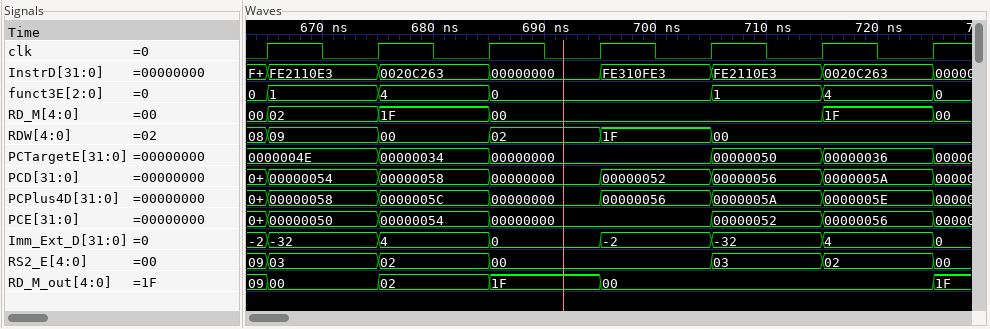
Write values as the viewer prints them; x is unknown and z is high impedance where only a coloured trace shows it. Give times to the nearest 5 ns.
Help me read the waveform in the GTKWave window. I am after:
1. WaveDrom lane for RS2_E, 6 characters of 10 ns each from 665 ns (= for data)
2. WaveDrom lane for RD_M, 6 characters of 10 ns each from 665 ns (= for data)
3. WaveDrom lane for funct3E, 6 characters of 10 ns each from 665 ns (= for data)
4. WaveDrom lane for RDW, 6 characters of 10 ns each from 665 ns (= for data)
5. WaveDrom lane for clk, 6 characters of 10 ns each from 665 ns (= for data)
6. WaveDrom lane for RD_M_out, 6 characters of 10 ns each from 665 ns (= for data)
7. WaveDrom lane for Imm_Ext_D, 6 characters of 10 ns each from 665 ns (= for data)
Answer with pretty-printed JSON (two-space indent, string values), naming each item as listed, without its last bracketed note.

{
  "WaveDrom lane for RS2_E, 6 characters of 10 ns each from 665 ns": "{name: 'RS2_E', wave: '===.==', data: '03 02 00 03 02'}",
  "WaveDrom lane for RD_M, 6 characters of 10 ns each from 665 ns": "{name: 'RD_M', wave: '===..=', data: '02 1F 00 1F'}",
  "WaveDrom lane for funct3E, 6 characters of 10 ns each from 665 ns": "{name: 'funct3E', wave: '===.==', data: '1 4 0 1 4'}",
  "WaveDrom lane for RDW, 6 characters of 10 ns each from 665 ns": "{name: 'RDW', wave: '=====.', data: '09 00 02 1F 00'}",
  "WaveDrom lane for clk, 6 characters of 10 ns each from 665 ns": "{name: 'clk', wave: 'p.....'}",
  "WaveDrom lane for RD_M_out, 6 characters of 10 ns each from 665 ns": "{name: 'RD_M_out', wave: '====..', data: '00 02 1F 00'}",
  "WaveDrom lane for Imm_Ext_D, 6 characters of 10 ns each from 665 ns": "{name: 'Imm_Ext_D', wave: '======', data: '-32 4 0 -2 -32 4'}"
}
